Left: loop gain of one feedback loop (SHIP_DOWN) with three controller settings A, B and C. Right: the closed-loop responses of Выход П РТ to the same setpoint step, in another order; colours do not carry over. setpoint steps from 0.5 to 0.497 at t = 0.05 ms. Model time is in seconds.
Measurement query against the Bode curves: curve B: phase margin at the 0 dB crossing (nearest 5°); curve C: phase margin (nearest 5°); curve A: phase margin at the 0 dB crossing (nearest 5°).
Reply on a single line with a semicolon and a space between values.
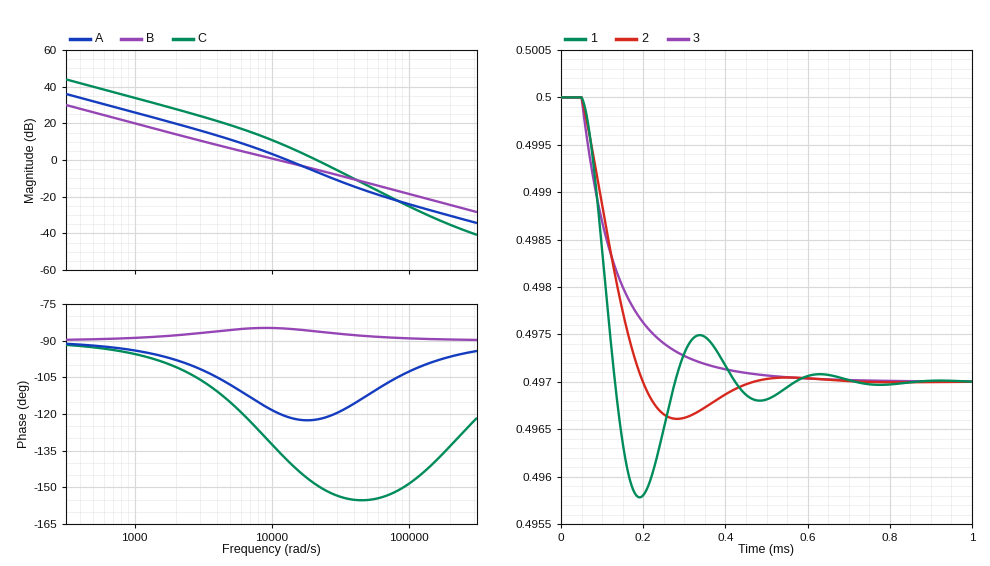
95°; 30°; 60°
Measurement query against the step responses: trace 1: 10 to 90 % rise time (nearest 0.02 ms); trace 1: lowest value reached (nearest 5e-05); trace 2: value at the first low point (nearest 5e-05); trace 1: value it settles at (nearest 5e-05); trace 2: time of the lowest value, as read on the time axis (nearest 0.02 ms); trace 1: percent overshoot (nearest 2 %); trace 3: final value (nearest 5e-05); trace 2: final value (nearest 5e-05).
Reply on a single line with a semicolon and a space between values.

0.06 ms; 0.49580; 0.49660; 0.49700; 0.28 ms; 40 %; 0.49700; 0.49700
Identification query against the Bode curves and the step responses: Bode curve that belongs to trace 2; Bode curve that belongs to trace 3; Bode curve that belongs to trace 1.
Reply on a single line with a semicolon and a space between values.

A; B; C
